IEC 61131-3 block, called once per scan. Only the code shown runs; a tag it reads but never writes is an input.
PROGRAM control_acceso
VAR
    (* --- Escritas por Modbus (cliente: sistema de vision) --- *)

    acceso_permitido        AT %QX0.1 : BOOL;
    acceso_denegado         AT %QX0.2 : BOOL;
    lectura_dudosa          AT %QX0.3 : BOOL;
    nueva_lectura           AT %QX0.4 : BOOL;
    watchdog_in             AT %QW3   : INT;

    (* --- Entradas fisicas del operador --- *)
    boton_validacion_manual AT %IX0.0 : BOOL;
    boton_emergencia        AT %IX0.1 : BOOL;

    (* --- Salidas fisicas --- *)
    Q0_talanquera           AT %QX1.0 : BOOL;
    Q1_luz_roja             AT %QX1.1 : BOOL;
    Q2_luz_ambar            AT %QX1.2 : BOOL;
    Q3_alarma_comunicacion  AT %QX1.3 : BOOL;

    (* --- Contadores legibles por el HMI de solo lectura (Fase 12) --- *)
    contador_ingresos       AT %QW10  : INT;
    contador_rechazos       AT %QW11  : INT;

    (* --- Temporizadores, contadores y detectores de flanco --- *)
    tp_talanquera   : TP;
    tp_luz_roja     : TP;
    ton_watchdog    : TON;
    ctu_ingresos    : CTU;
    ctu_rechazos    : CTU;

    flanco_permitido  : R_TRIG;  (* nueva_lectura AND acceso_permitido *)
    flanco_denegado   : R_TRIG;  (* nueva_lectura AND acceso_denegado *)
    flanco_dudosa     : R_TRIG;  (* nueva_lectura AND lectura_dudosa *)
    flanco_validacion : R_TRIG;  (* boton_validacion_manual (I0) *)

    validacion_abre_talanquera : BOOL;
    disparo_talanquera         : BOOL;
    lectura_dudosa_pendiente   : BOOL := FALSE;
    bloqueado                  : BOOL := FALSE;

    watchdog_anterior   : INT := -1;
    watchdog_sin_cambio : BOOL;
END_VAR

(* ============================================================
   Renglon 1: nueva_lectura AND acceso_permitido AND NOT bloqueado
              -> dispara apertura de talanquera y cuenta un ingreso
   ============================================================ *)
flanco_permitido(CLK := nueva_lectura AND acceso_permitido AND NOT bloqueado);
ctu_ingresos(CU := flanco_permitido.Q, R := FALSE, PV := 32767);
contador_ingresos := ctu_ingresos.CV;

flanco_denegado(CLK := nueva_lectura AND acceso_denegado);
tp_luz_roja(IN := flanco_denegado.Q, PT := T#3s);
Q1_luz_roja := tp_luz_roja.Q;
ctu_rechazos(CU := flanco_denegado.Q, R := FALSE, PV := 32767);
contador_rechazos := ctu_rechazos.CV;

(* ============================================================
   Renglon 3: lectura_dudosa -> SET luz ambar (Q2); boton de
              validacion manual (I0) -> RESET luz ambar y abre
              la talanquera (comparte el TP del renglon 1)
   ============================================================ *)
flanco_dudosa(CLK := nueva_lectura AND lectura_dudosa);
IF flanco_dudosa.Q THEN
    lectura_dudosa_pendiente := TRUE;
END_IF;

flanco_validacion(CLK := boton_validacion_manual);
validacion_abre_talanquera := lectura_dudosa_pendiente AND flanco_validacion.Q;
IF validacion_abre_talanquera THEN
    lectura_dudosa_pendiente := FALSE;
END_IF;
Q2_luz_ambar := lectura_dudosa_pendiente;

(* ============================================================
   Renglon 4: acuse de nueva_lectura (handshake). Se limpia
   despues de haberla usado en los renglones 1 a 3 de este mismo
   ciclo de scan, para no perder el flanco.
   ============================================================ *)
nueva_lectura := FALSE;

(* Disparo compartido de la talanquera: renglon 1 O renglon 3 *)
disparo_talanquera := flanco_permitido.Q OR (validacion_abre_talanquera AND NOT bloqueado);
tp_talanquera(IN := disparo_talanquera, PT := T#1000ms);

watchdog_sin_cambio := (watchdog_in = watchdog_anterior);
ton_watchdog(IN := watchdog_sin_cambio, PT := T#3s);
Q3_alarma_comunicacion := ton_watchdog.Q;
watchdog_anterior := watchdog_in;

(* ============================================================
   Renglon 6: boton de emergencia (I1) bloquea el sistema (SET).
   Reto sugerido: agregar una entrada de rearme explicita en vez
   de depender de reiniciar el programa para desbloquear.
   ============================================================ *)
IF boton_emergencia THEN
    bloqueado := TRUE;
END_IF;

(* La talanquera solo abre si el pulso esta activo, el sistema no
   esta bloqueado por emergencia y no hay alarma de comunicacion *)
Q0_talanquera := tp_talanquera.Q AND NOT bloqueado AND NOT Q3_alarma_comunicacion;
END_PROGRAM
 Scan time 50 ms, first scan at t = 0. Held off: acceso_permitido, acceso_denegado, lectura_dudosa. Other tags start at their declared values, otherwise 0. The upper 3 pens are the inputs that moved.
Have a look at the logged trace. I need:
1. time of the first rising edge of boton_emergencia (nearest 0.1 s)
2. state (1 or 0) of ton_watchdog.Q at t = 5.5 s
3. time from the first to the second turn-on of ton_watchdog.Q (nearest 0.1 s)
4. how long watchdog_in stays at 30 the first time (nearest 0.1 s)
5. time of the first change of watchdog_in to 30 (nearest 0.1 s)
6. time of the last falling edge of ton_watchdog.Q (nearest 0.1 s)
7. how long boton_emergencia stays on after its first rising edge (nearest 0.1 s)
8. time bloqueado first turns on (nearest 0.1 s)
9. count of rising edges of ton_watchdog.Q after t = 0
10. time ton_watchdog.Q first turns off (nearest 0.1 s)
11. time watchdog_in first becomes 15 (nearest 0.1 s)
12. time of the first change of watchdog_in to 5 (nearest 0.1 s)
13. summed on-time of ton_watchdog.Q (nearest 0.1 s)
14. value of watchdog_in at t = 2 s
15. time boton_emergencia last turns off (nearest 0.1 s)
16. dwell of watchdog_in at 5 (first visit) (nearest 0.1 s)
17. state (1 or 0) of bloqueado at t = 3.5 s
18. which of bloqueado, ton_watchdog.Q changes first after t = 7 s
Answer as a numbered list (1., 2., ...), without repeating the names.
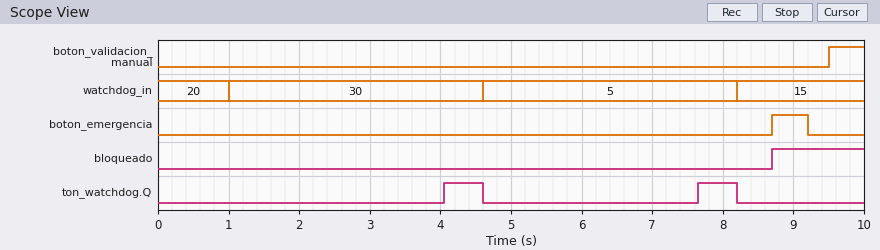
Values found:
1. 8.7 s
2. 0
3. 3.6 s
4. 3.6 s
5. 1.0 s
6. 8.2 s
7. 0.5 s
8. 8.7 s
9. 2
10. 4.6 s
11. 8.2 s
12. 4.6 s
13. 1.1 s
14. 30
15. 9.2 s
16. 3.6 s
17. 0
18. ton_watchdog.Q
